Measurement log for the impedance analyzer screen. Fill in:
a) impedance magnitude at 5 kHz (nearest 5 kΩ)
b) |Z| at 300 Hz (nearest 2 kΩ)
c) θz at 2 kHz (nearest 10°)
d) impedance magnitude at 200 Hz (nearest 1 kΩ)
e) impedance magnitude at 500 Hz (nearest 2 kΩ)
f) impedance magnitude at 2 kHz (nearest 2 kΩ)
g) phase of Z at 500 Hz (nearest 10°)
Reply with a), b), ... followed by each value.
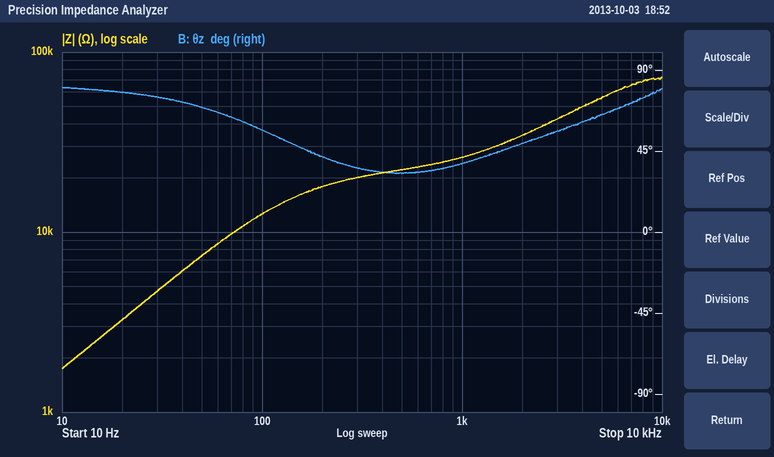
a) 55 kΩ
b) 20 kΩ
c) 50°
d) 18 kΩ
e) 22 kΩ
f) 34 kΩ
g) 30°
